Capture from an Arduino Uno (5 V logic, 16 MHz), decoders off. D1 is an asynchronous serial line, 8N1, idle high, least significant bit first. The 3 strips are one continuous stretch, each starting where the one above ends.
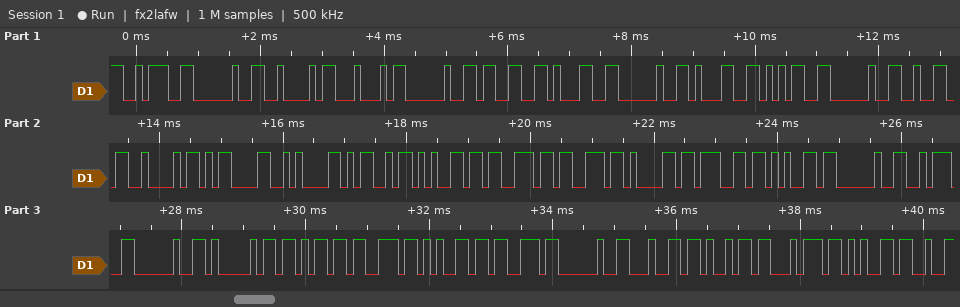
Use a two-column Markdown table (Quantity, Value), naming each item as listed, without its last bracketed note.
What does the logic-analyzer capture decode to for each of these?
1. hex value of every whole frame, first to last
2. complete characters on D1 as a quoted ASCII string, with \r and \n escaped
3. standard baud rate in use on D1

| Quantity | Value |
|---|---|
| hex value of every whole frame, first to last | 3A 20 42 44 20 33 31 20 31 35 20 32 42 0D 0A 4D 65 73 73 61 67 65 20 3A 20 41 6B 73 65 73 20 64 69 74 65 |
| complete characters on D1 as a quoted ASCII string, with \r and \n escaped | ": BD 31 15 2B\r\nMessage : Akses dite" |
| standard baud rate in use on D1 | 9600 baud |
